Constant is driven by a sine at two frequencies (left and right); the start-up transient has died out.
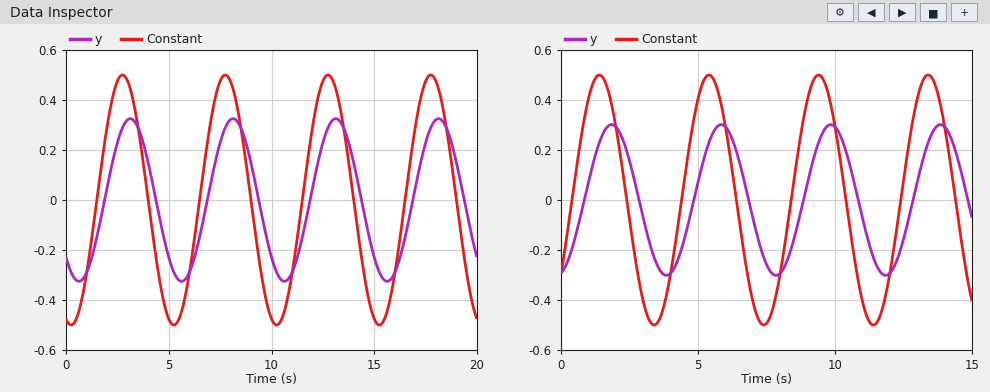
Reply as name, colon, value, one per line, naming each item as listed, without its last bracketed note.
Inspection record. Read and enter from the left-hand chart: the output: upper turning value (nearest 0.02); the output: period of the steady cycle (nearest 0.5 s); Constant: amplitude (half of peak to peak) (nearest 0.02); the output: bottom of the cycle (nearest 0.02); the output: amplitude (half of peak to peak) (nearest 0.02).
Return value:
the output: upper turning value: 0.32
the output: period of the steady cycle: 5.0 s
Constant: amplitude (half of peak to peak): 0.50
the output: bottom of the cycle: -0.32
the output: amplitude (half of peak to peak): 0.32
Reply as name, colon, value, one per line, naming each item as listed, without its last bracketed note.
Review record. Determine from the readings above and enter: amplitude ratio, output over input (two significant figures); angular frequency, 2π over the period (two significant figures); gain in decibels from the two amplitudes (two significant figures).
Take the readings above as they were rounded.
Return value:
amplitude ratio, output over input: 0.64
angular frequency, 2π over the period: 1.3 rad/s
gain in decibels from the two amplitudes: -3.9 dB
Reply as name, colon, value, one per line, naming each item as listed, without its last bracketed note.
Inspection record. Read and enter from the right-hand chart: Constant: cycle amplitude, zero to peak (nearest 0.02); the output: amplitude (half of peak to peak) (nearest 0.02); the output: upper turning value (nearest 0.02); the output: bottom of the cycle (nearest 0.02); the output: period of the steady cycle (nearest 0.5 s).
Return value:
Constant: cycle amplitude, zero to peak: 0.50
the output: amplitude (half of peak to peak): 0.30
the output: upper turning value: 0.30
the output: bottom of the cycle: -0.30
the output: period of the steady cycle: 4.0 s
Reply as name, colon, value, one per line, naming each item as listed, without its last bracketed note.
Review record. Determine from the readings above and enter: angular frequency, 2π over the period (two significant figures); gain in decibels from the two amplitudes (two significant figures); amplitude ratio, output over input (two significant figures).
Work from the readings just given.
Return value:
angular frequency, 2π over the period: 1.6 rad/s
gain in decibels from the two amplitudes: -4.4 dB
amplitude ratio, output over input: 0.60
